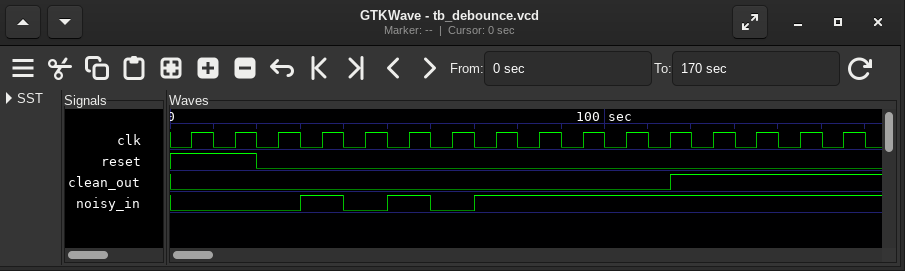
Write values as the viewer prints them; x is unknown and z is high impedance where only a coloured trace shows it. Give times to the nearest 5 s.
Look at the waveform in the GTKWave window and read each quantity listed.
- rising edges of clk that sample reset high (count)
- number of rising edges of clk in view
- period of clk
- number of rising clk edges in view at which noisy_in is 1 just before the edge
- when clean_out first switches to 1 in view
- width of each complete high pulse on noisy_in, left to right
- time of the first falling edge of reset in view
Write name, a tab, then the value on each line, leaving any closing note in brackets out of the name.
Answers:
rising edges of clk that sample reset high	2
number of rising edges of clk in view	16
period of clk	10 s
number of rising clk edges in view at which noisy_in is 1 just before the edge	11
when clean_out first switches to 1 in view	115 s
width of each complete high pulse on noisy_in, left to right	10 s, 10 s
time of the first falling edge of reset in view	20 s
